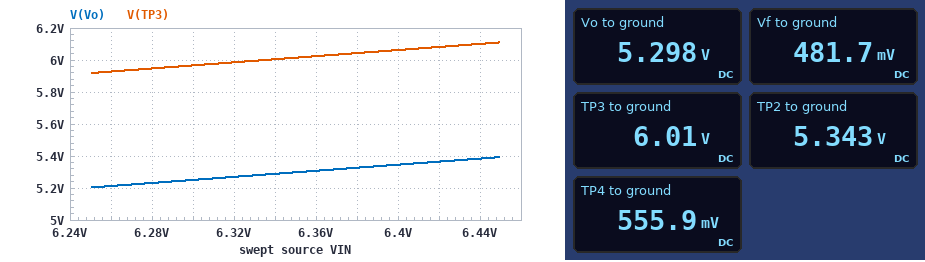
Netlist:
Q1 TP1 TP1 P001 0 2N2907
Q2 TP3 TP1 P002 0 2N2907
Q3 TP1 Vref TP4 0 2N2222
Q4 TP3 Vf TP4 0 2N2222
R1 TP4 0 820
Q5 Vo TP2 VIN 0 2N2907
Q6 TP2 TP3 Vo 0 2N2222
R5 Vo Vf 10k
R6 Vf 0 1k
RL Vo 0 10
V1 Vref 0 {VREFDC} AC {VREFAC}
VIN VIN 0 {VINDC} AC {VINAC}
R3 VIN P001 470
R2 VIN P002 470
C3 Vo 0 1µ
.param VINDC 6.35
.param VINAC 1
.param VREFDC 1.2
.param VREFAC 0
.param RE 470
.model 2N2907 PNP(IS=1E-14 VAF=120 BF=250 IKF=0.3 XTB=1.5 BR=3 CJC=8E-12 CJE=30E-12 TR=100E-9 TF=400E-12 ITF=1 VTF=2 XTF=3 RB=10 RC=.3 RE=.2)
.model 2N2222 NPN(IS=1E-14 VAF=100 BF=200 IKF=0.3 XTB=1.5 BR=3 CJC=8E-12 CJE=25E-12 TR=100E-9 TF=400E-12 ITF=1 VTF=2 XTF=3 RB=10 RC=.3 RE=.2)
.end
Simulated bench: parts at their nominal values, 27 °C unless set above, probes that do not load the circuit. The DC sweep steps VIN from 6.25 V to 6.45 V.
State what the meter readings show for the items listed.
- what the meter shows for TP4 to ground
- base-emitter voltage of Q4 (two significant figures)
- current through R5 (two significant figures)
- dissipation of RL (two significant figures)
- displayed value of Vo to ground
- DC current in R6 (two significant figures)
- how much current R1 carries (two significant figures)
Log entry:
555.9 mV
-74 mV
480 µA
2.8 W
5.298 V
480 µA
680 µA
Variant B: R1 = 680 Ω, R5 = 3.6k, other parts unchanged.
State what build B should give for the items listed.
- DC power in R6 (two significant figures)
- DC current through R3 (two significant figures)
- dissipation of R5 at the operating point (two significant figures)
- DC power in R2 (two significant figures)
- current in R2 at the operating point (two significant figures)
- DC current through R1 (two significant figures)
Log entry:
1.3 mW
650 µA
4.8 mW
190 µW
640 µA
820 µA
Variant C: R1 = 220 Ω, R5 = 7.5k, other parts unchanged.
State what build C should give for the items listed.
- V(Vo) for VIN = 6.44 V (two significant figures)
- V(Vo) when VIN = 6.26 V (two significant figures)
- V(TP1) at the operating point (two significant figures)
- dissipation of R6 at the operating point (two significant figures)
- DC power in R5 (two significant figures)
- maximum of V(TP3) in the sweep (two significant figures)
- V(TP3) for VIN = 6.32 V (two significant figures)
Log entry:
5.2 V
5.0 V
5.1 V
360 µW
2.7 mW
5.9 V
5.8 V
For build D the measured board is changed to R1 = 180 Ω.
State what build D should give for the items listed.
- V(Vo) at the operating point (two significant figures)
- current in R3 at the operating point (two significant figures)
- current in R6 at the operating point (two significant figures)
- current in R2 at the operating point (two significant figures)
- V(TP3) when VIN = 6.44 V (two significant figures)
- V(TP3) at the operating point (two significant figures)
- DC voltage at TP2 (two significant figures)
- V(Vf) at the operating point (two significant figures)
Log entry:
5.0 V
1.5 mA
450 µA
1.4 mA
5.8 V
5.7 V
5.4 V
450 mV
